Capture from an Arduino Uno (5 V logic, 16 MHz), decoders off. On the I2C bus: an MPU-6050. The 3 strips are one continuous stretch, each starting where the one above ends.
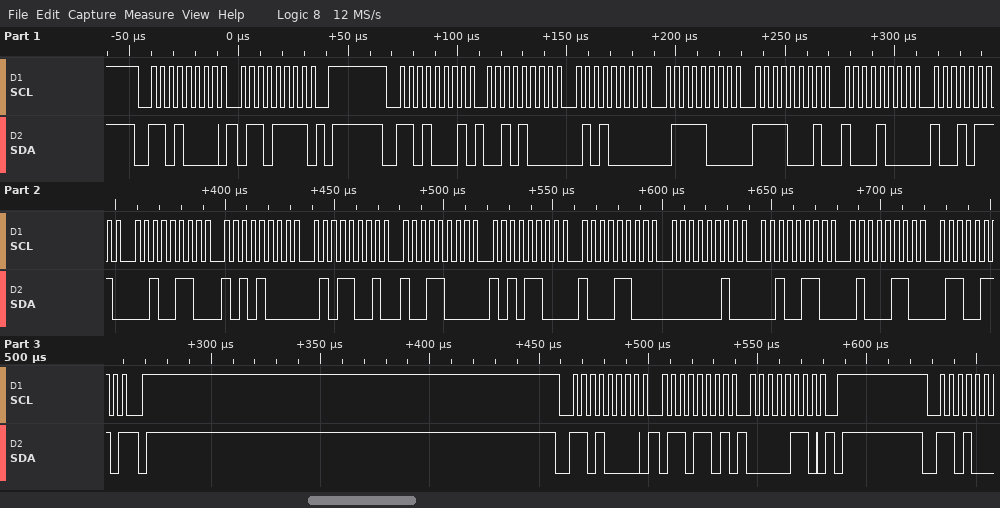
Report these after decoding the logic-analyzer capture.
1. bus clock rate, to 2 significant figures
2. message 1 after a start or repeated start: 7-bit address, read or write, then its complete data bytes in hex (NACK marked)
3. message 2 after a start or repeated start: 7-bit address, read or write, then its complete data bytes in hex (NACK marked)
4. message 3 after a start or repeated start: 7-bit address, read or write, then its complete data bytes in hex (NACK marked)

250 kHz
0x68 write: 6F
0x68 read: 28 50 78 F1 88 97 26 A8 59 98 AC 8C 02 26 46 66 NACK
0x68 write: 6D 06
